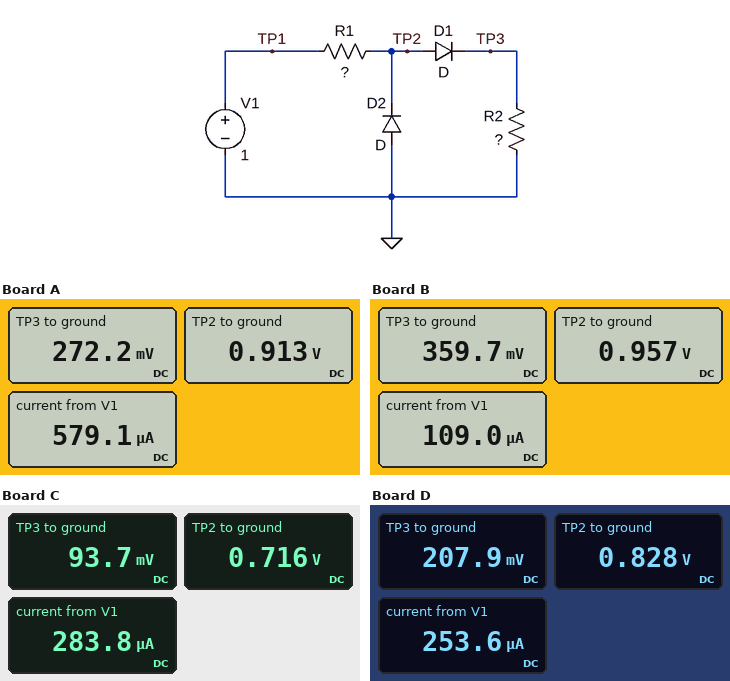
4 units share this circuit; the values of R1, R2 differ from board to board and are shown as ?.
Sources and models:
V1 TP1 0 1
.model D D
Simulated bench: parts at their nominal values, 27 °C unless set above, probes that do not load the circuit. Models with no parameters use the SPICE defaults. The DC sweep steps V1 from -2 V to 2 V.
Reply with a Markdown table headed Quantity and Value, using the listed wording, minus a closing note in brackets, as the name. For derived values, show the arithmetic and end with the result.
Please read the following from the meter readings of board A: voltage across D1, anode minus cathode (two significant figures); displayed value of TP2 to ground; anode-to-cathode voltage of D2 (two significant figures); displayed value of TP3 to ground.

| Quantity | Value |
|---|---|
| voltage across D1, anode minus cathode | 913 mV - 272.2 mV = 640 mV |
| displayed value of TP2 to ground | 0.913 V |
| anode-to-cathode voltage of D2 | 0 V - 913 mV = -910 mV |
| displayed value of TP3 to ground | 272.2 mV |
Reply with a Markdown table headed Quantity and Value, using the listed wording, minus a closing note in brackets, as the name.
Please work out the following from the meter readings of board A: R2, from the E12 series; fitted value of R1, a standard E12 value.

| Quantity | Value |
|---|---|
| R2, from the E12 series | 470 Ω |
| fitted value of R1, a standard E12 value | 150 Ω |
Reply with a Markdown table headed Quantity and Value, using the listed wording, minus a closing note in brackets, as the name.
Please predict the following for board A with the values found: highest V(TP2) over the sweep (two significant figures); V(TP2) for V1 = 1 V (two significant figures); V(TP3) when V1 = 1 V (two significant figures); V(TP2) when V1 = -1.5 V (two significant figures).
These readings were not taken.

| Quantity | Value |
|---|---|
| highest V(TP2) over the sweep | 1.7 V |
| V(TP2) for V1 = 1 V | 910 mV |
| V(TP3) when V1 = 1 V | 270 mV |
| V(TP2) when V1 = -1.5 V | -700 mV |
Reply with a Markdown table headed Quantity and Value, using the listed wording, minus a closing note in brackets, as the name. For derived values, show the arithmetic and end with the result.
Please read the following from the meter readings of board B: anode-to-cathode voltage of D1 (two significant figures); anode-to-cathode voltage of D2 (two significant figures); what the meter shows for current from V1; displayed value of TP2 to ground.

| Quantity | Value |
|---|---|
| anode-to-cathode voltage of D1 | 957 mV - 359.7 mV = 600 mV |
| anode-to-cathode voltage of D2 | 0 V - 957 mV = -960 mV |
| what the meter shows for current from V1 | 109.0 µA |
| displayed value of TP2 to ground | 0.957 V |
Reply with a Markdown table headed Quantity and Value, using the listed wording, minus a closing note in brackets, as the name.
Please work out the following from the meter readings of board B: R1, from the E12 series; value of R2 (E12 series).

| Quantity | Value |
|---|---|
| R1, from the E12 series | 390 Ω |
| value of R2 | 3.3 kΩ |
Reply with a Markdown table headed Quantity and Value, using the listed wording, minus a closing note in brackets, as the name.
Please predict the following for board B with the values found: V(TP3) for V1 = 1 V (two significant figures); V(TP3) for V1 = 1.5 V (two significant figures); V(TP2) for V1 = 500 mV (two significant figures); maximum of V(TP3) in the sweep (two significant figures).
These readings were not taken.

| Quantity | Value |
|---|---|
| V(TP3) for V1 = 1 V | 360 mV |
| V(TP3) for V1 = 1.5 V | 790 mV |
| V(TP2) for V1 = 500 mV | 500 mV |
| maximum of V(TP3) in the sweep | 1.2 V |
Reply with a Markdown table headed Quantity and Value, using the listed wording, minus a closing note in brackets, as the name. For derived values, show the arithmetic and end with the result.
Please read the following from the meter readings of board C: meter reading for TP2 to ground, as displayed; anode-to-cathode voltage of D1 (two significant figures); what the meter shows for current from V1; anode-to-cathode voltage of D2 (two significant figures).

| Quantity | Value |
|---|---|
| meter reading for TP2 to ground, as displayed | 0.716 V |
| anode-to-cathode voltage of D1 | 716 mV - 93.7 mV = 620 mV |
| what the meter shows for current from V1 | 283.8 µA |
| anode-to-cathode voltage of D2 | 0 V - 716 mV = -720 mV |
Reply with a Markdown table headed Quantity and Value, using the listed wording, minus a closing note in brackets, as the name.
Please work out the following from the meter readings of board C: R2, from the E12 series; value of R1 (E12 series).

| Quantity | Value |
|---|---|
| R2, from the E12 series | 330 Ω |
| value of R1 | 1 kΩ |
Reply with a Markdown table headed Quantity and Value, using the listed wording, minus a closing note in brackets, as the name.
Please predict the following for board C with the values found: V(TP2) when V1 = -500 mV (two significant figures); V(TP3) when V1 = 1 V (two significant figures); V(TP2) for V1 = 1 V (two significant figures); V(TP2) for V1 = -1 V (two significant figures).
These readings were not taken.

| Quantity | Value |
|---|---|
| V(TP2) when V1 = -500 mV | -500 mV |
| V(TP3) when V1 = 1 V | 94 mV |
| V(TP2) for V1 = 1 V | 720 mV |
| V(TP2) for V1 = -1 V | -630 mV |
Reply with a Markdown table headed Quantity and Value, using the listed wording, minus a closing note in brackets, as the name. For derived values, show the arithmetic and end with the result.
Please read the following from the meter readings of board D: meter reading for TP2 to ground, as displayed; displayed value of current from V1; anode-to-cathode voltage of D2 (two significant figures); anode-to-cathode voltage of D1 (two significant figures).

| Quantity | Value |
|---|---|
| meter reading for TP2 to ground, as displayed | 0.828 V |
| displayed value of current from V1 | 253.6 µA |
| anode-to-cathode voltage of D2 | 0 V - 828 mV = -830 mV |
| anode-to-cathode voltage of D1 | 828 mV - 207.9 mV = 620 mV |
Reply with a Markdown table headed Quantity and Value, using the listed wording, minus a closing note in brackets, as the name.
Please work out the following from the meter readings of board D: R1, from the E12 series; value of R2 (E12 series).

| Quantity | Value |
|---|---|
| R1, from the E12 series | 680 Ω |
| value of R2 | 820 Ω |
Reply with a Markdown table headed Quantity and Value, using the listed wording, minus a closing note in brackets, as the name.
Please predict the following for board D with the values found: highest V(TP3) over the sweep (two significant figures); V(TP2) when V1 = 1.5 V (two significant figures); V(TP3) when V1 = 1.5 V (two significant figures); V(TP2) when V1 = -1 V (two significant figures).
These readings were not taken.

| Quantity | Value |
|---|---|
| highest V(TP3) over the sweep | 740 mV |
| V(TP2) when V1 = 1.5 V | 1.1 V |
| V(TP3) when V1 = 1.5 V | 470 mV |
| V(TP2) when V1 = -1 V | -640 mV |
